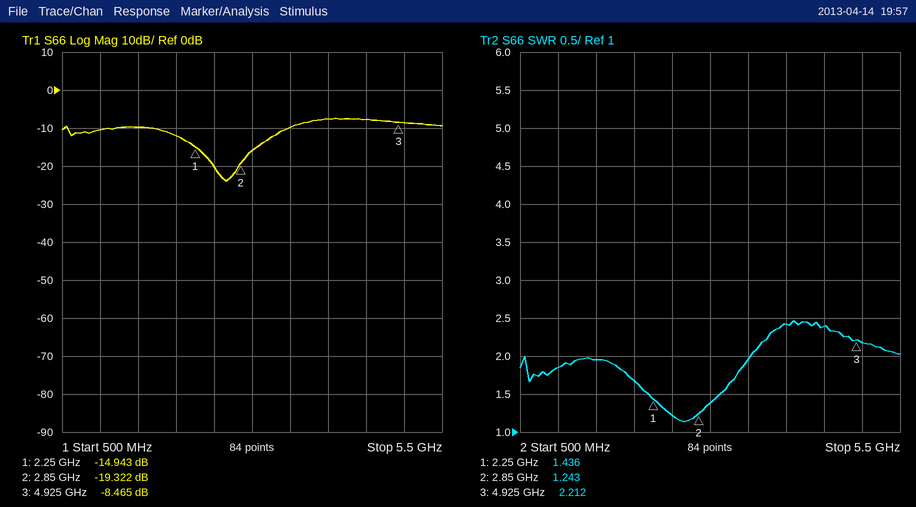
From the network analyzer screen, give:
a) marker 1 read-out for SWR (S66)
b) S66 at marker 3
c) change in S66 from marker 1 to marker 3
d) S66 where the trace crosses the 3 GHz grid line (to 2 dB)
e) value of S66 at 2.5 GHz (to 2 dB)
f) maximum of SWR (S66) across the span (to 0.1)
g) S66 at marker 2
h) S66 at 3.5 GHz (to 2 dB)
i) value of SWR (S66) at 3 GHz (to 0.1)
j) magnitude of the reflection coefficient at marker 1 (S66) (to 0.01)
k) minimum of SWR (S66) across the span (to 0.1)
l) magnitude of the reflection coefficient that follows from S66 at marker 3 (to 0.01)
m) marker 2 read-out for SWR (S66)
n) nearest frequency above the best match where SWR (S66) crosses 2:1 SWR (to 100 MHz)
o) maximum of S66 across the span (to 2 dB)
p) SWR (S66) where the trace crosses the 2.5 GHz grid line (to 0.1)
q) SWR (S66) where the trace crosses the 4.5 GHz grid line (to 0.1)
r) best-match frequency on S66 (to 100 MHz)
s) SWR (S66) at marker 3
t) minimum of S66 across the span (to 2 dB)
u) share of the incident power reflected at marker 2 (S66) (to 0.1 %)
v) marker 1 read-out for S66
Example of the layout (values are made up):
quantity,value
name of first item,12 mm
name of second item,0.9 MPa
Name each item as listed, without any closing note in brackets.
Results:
quantity,value
marker 1 read-out for SWR,1.436
S66 at marker 3,-8.465 dB
change in S66 from marker 1 to marker 3,6.478 dB
S66 where the trace crosses the 3 GHz grid line,-16 dB
value of S66 at 2.5 GHz,-20 dB
maximum of SWR (S66) across the span,2.5
S66 at marker 2,-19.322 dB
S66 at 3.5 GHz,-10 dB
value of SWR (S66) at 3 GHz,1.4
magnitude of the reflection coefficient at marker 1 (S66),0.18
minimum of SWR (S66) across the span,1.1
magnitude of the reflection coefficient that follows from S66 at marker 3,0.38
marker 2 read-out for SWR,1.243
nearest frequency above the best match where SWR (S66) crosses 2:1 SWR,3.5 GHz
maximum of S66 across the span,-8 dB
SWR (S66) where the trace crosses the 2.5 GHz grid line,1.2
SWR (S66) where the trace crosses the 4.5 GHz grid line,2.4
best-match frequency on S66,2.7 GHz
SWR (S66) at marker 3,2.212
minimum of S66 across the span,-24 dB
share of the incident power reflected at marker 2 (S66),1.2 %
marker 1 read-out for S66,-14.943 dB
